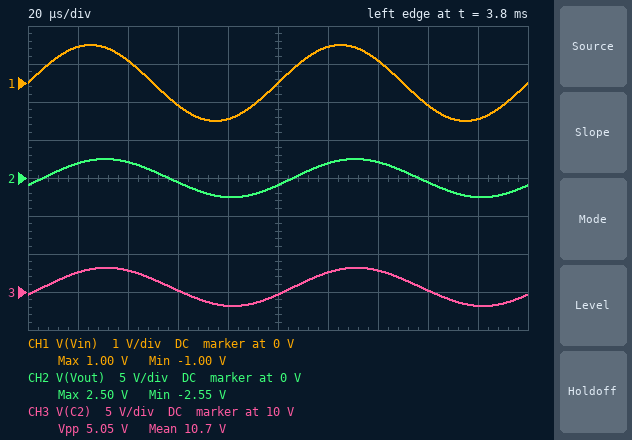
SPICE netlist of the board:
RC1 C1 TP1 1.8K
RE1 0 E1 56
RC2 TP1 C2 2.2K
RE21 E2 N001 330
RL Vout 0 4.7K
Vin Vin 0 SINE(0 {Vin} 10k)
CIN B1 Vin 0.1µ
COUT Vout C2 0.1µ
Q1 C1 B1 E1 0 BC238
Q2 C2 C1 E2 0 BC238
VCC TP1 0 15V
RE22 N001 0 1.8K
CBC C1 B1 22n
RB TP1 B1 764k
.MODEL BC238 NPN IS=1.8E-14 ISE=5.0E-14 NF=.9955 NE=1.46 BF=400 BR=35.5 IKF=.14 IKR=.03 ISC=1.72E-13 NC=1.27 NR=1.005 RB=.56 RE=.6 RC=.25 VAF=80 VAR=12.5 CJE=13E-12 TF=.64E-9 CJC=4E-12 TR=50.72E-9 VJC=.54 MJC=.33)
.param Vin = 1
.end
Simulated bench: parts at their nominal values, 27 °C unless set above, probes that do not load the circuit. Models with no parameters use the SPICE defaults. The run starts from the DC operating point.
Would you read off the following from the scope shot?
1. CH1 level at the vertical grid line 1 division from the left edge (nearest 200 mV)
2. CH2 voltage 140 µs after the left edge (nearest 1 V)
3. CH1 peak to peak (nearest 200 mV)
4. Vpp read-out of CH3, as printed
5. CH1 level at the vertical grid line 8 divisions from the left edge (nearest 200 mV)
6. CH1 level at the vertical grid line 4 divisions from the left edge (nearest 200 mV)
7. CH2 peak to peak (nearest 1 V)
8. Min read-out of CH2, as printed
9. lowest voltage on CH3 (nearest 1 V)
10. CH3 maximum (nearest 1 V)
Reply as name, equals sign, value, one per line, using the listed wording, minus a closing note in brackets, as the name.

CH1 level at the vertical grid line 1 division from the left edge = 1.0 V
CH2 voltage 140 µs after the left edge = 2 V
CH1 peak to peak = 2.0 V
Vpp read-out of CH3, as printed = 5.05 V
CH1 level at the vertical grid line 8 divisions from the left edge = -600 mV
CH1 level at the vertical grid line 4 divisions from the left edge = -1.0 V
CH2 peak to peak = 5 V
Min read-out of CH2, as printed = -2.55 V
lowest voltage on CH3 = 8 V
CH3 maximum = 13 V
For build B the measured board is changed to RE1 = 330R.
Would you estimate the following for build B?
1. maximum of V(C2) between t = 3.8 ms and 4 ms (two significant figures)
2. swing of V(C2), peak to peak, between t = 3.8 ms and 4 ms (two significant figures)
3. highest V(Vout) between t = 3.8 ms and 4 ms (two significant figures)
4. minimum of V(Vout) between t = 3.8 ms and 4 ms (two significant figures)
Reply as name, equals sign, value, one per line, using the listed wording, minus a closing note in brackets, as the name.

maximum of V(C2) between t = 3.8 ms and 4 ms = 11 V
swing of V(C2), peak to peak, between t = 3.8 ms and 4 ms = 2.4 V
highest V(Vout) between t = 3.8 ms and 4 ms = 1.2 V
minimum of V(Vout) between t = 3.8 ms and 4 ms = -1.2 V
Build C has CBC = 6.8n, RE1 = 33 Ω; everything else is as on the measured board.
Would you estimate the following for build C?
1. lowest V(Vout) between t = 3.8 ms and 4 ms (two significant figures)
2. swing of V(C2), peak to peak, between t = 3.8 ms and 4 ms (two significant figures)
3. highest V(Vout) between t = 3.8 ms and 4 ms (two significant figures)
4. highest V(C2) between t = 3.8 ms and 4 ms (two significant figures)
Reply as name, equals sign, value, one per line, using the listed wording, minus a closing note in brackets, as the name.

lowest V(Vout) between t = 3.8 ms and 4 ms = -2.8 V
swing of V(C2), peak to peak, between t = 3.8 ms and 4 ms = 5.9 V
highest V(Vout) between t = 3.8 ms and 4 ms = 3.0 V
highest V(C2) between t = 3.8 ms and 4 ms = 14 V
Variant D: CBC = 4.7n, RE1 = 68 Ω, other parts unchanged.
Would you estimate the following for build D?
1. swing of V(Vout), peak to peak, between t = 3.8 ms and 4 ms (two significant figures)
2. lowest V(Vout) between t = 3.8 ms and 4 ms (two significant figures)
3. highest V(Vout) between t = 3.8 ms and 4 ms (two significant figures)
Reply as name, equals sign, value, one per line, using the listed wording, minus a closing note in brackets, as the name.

swing of V(Vout), peak to peak, between t = 3.8 ms and 4 ms = 5.7 V
lowest V(Vout) between t = 3.8 ms and 4 ms = -2.7 V
highest V(Vout) between t = 3.8 ms and 4 ms = 3.0 V
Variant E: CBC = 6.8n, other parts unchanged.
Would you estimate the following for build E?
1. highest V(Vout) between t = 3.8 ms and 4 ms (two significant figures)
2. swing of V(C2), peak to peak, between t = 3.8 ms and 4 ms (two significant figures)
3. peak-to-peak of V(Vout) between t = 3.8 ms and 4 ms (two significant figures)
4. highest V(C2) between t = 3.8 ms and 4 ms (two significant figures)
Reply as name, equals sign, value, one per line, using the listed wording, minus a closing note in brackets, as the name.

highest V(Vout) between t = 3.8 ms and 4 ms = 3.0 V
swing of V(C2), peak to peak, between t = 3.8 ms and 4 ms = 5.8 V
peak-to-peak of V(Vout) between t = 3.8 ms and 4 ms = 5.7 V
highest V(C2) between t = 3.8 ms and 4 ms = 14 V
